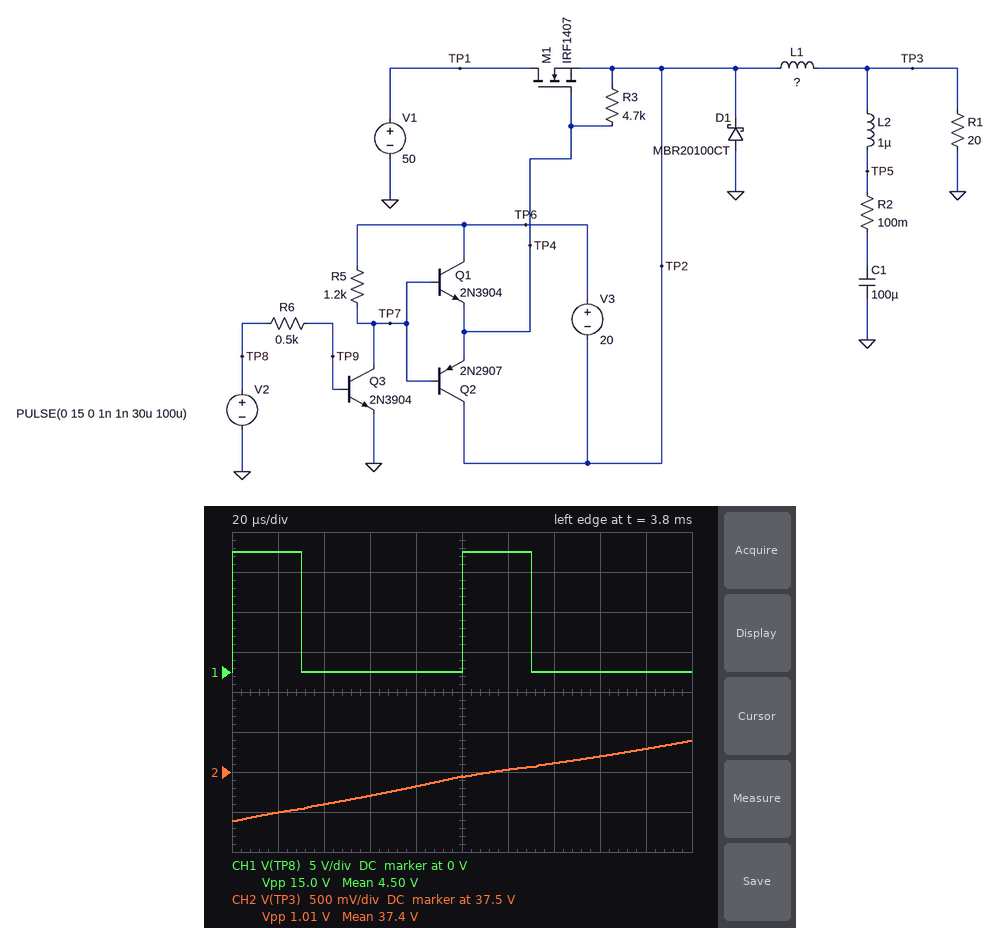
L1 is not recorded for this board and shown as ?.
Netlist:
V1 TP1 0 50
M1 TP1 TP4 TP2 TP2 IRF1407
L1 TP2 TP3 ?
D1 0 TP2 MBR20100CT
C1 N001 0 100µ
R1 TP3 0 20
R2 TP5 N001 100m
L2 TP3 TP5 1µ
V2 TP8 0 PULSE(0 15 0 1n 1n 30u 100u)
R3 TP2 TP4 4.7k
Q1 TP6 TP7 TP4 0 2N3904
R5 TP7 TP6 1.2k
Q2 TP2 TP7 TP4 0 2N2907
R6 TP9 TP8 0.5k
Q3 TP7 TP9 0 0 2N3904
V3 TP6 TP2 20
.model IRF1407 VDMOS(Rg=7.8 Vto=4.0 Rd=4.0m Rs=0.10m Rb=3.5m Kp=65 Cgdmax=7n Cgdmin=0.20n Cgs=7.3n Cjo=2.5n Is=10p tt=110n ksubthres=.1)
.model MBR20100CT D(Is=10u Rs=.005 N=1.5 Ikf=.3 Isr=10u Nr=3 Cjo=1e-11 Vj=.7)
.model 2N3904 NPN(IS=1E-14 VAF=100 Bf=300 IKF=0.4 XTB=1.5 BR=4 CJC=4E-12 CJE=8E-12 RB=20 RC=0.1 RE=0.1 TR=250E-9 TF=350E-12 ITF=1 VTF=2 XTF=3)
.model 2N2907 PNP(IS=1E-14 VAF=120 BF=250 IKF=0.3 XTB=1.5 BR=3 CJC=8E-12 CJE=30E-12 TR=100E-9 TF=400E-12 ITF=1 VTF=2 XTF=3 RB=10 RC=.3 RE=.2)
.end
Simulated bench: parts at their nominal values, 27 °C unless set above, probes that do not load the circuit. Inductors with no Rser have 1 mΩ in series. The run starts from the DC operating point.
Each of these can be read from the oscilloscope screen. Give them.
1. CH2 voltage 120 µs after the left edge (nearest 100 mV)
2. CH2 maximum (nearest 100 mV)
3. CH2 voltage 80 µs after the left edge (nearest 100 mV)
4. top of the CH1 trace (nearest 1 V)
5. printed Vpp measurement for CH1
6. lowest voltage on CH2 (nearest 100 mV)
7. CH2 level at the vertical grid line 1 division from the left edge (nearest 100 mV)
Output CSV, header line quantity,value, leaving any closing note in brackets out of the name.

quantity,value
CH2 voltage 120 µs after the left edge,37.5 V
CH2 maximum,37.9 V
CH2 voltage 80 µs after the left edge,37.3 V
top of the CH1 trace,15 V
printed Vpp measurement for CH1,15.0 V
lowest voltage on CH2,36.9 V
CH2 level at the vertical grid line 1 division from the left edge,37.0 V
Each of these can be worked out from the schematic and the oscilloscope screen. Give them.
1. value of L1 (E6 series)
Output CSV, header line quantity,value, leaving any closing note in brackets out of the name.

quantity,value
value of L1,4.7 mH
